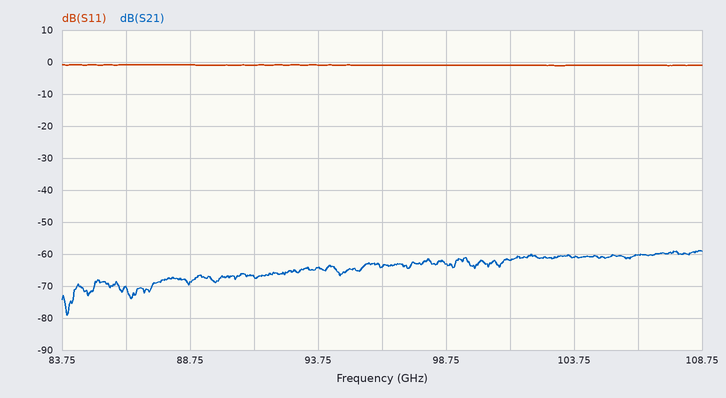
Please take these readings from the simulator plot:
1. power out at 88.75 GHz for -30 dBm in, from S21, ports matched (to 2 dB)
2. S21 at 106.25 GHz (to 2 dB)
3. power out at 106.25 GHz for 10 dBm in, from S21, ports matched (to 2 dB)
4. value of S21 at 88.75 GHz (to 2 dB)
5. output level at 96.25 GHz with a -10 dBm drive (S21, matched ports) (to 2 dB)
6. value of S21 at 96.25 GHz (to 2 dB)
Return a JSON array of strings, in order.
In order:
["-98 dBm", "-60 dB", "-50 dBm", "-68 dB", "-74 dBm", "-64 dB"]
